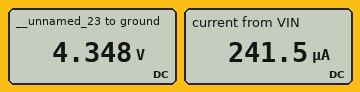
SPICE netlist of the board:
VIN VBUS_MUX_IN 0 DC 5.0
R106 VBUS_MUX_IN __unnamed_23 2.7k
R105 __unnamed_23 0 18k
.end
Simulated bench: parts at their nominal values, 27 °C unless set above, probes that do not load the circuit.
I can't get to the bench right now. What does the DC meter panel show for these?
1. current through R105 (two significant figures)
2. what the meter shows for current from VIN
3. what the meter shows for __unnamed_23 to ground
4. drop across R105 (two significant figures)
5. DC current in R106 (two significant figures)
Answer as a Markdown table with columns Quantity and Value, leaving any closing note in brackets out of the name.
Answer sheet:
| Quantity | Value |
|---|---|
| current through R105 | 240 µA |
| what the meter shows for current from VIN | 241.5 µA |
| what the meter shows for __unnamed_23 to ground | 4.348 V |
| drop across R105 | 4.3 V |
| DC current in R106 | 240 µA |
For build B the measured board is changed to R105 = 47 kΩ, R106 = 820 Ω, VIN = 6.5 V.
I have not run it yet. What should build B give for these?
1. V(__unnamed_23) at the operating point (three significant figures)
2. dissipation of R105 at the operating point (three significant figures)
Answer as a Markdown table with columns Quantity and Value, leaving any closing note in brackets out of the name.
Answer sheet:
| Quantity | Value |
|---|---|
| V(__unnamed_23) at the operating point | 6.39 V |
| dissipation of R105 at the operating point | 868 µW |
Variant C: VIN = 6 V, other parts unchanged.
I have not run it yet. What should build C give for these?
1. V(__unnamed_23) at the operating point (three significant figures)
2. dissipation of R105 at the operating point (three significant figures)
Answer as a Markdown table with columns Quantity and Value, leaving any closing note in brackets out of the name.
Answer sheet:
| Quantity | Value |
|---|---|
| V(__unnamed_23) at the operating point | 5.22 V |
| dissipation of R105 at the operating point | 1.51 mW |
